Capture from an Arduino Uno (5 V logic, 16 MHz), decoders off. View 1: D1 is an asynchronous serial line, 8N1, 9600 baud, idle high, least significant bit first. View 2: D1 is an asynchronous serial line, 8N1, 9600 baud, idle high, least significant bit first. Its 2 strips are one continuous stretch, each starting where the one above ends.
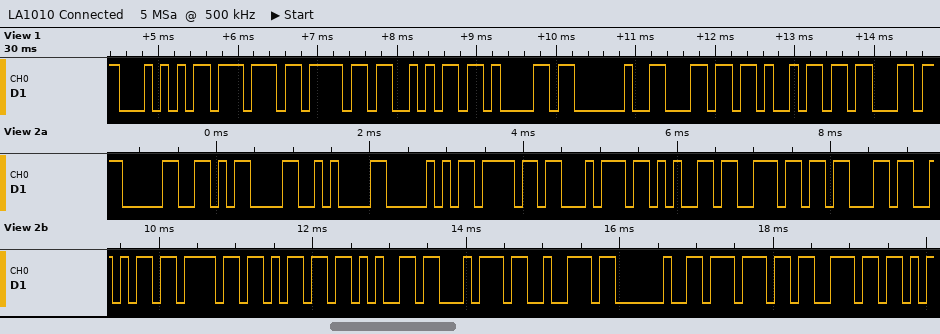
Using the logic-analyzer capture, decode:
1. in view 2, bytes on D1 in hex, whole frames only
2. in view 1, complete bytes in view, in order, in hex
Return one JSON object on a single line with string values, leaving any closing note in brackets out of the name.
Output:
{"in view 2, bytes on D1 in hex, whole frames only": "0x30 0x0D 0x0A 0x50 0x6F 0x74 0x65 0x6E 0x63 0x6A 0x6F 0x6D 0x65 0x74 0x72 0x20 0x77 0x73", "in view 1, complete bytes in view, in order, in hex": "0x54 0x77 0x6F 0x6A 0x61 0x20 0x6C 0x69 0x63"}
